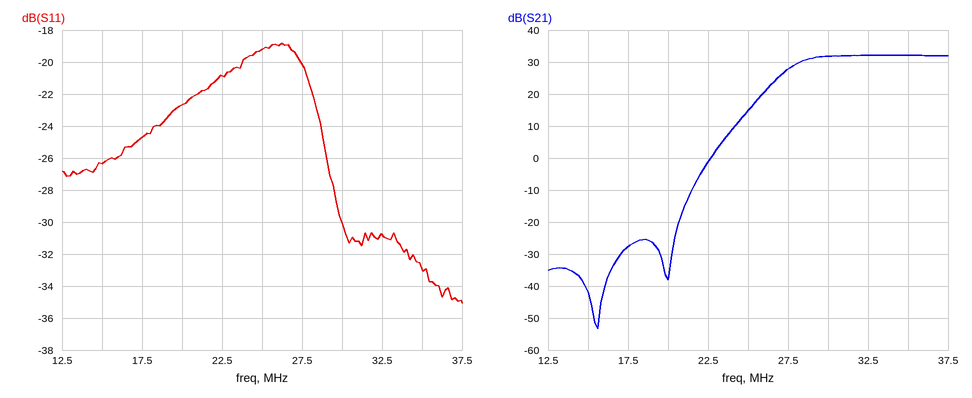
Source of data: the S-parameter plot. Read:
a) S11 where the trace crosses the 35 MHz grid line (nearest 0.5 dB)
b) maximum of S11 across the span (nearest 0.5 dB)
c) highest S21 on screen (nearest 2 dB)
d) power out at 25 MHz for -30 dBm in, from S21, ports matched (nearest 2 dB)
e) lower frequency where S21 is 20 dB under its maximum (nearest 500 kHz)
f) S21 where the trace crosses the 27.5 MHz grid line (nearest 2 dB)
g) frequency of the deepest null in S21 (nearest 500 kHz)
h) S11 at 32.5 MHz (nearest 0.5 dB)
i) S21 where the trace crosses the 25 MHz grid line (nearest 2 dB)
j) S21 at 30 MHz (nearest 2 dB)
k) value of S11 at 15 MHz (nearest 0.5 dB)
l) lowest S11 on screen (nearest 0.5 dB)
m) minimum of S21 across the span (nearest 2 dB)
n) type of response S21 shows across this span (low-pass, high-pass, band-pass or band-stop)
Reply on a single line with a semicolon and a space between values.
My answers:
-33.0 dB; -19.0 dB; 32 dB; -16 dBm; 24.5 MHz; 28 dB; 15.5 MHz; -31.0 dB; 14 dB; 32 dB; -26.5 dB; -35.0 dB; -54 dB; high-pass
